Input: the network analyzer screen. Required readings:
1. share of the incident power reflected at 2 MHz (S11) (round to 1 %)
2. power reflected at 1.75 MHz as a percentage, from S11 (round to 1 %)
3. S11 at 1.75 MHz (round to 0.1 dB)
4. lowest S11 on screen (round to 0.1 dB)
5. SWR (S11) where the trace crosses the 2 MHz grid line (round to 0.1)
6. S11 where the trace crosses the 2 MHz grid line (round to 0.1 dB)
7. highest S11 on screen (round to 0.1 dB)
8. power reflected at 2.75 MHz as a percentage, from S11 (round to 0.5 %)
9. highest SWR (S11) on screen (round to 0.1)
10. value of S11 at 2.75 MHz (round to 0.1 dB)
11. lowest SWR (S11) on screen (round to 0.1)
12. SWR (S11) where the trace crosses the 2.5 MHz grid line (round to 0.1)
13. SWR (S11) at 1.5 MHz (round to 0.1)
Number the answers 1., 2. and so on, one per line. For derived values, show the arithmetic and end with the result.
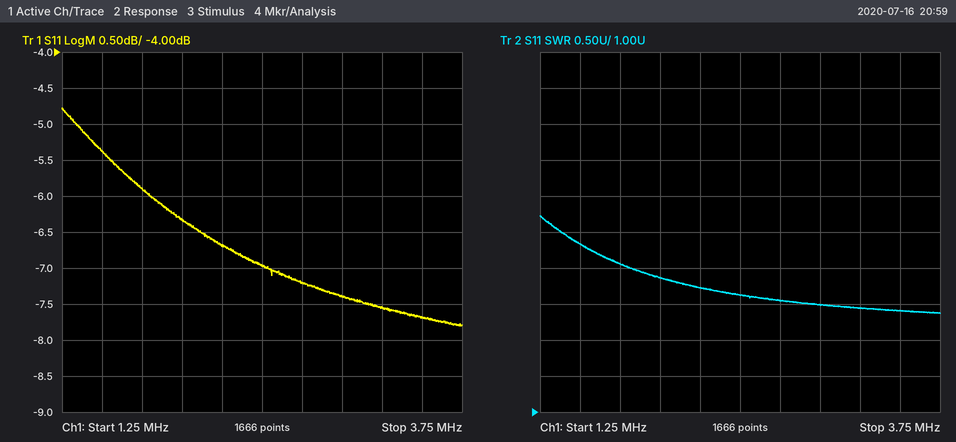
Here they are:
1. 10^(-6.3/10) ≈ 23 %
2. 10^(-5.9/10) ≈ 26 %
3. -5.9 dB
4. -7.8 dB
5. 2.9
6. -6.3 dB
7. -4.8 dB
8. 10^(-7.2/10) ≈ 19.1 %, so 19.0 % to the nearest 0.5 %
9. 3.7
10. -7.2 dB
11. 2.4
12. 2.6
13. 3.3
